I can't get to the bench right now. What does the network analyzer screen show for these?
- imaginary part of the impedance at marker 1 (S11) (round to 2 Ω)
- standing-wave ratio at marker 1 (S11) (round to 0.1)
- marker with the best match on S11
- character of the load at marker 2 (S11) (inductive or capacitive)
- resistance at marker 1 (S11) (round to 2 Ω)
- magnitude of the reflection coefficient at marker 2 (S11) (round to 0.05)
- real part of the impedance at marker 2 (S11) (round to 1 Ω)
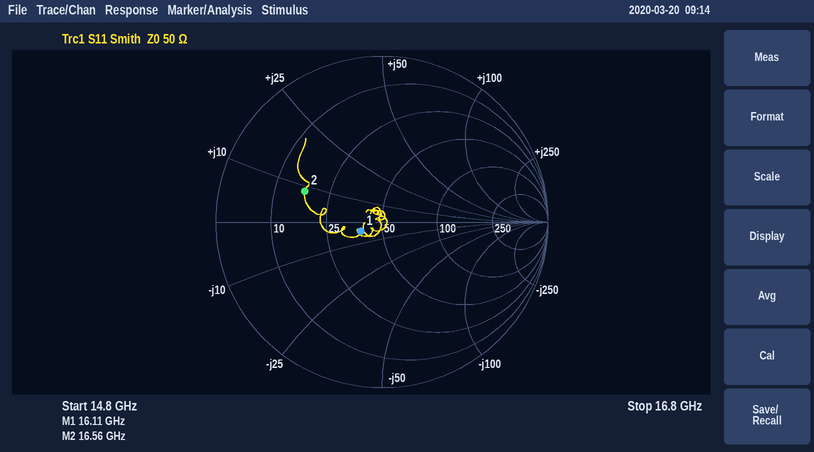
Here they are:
-4 Ω
1.3
marker 1
inductive
38 Ω
0.50
17 Ω
